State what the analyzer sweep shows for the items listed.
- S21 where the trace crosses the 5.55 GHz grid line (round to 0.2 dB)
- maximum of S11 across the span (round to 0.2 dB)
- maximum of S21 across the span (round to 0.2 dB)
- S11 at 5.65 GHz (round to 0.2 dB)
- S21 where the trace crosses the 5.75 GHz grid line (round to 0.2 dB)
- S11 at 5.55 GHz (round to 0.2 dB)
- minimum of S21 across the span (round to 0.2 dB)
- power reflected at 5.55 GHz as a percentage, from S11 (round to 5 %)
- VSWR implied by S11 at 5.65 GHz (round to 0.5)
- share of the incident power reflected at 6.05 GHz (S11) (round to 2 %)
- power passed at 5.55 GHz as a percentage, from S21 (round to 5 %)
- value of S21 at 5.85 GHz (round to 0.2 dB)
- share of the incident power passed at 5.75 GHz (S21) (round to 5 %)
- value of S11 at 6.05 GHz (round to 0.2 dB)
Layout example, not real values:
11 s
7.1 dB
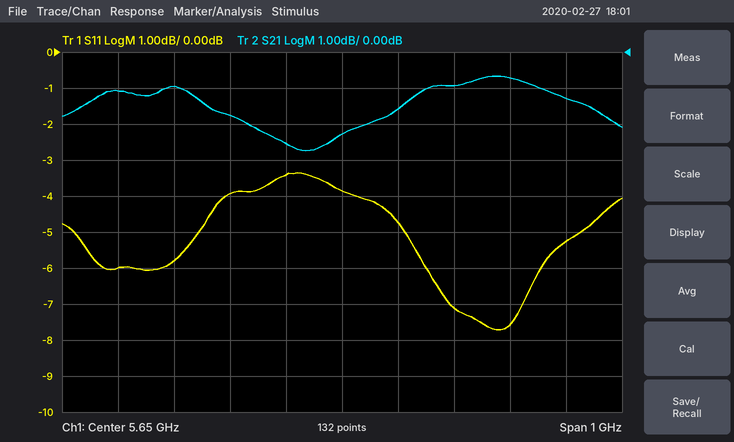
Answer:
-2.6 dB
-3.4 dB
-0.6 dB
-3.8 dB
-1.6 dB
-3.4 dB
-2.8 dB
45 %
4.5
30 %
55 %
-1.0 dB
70 %
-5.2 dB
